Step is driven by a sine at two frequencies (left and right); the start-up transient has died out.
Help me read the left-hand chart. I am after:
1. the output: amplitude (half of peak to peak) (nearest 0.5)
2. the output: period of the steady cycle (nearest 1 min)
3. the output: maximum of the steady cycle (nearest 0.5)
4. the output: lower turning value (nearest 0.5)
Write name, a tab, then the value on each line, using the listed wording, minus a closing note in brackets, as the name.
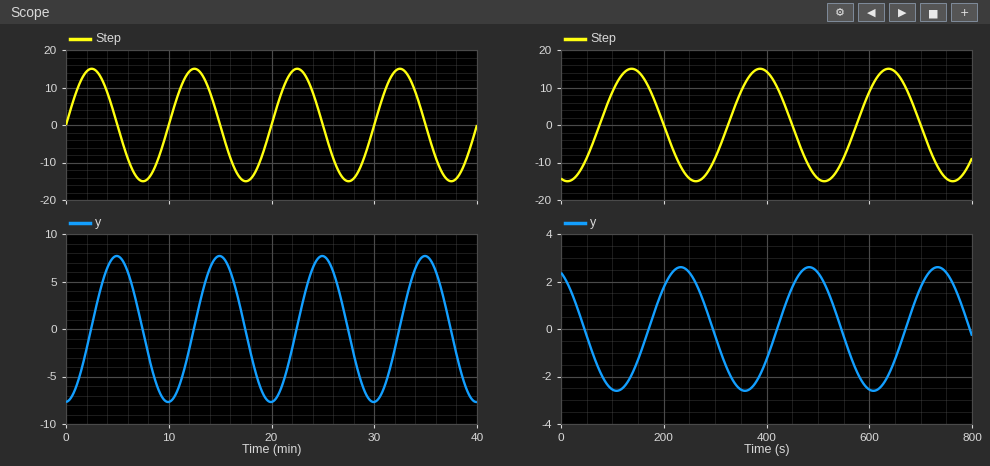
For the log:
the output: amplitude (half of peak to peak)	7.5
the output: period of the steady cycle	10 min
the output: maximum of the steady cycle	7.5
the output: lower turning value	-7.5
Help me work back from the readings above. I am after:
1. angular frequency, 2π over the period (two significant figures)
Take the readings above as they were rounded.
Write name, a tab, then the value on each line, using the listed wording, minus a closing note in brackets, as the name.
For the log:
angular frequency, 2π over the period	0.63 rad/min
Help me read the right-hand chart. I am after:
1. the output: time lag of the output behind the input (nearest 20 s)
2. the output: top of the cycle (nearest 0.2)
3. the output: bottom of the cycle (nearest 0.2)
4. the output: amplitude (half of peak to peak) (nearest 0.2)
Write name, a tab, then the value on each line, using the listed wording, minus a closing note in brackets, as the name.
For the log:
the output: time lag of the output behind the input	100 s
the output: top of the cycle	2.6
the output: bottom of the cycle	-2.6
the output: amplitude (half of peak to peak)	2.6
